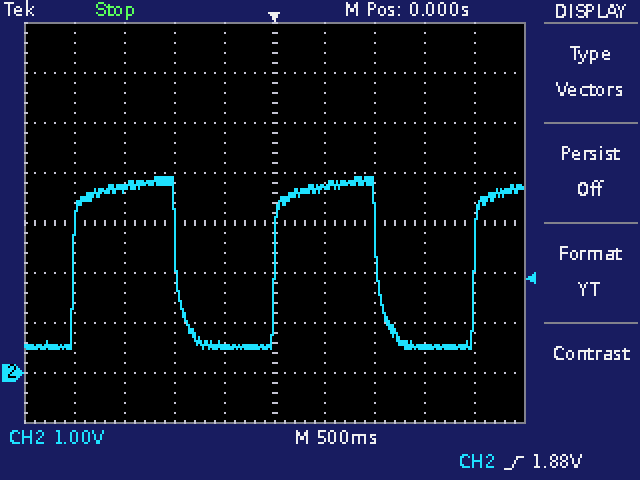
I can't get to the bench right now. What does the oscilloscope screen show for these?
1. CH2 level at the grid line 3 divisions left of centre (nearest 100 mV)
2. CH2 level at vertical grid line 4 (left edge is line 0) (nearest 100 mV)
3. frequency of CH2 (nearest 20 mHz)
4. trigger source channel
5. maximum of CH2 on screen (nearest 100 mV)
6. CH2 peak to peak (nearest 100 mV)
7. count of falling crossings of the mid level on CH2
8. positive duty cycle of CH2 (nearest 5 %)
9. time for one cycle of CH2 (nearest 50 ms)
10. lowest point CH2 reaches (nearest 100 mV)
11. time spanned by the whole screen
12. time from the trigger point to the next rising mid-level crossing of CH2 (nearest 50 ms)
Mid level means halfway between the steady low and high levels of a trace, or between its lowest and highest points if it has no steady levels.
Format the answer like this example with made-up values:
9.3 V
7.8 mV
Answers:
3.7 V
500 mV
500 mHz
CH2
3.9 V
3.4 V
2
50 %
2.00 s
500 mV
5 s
2.00 s
